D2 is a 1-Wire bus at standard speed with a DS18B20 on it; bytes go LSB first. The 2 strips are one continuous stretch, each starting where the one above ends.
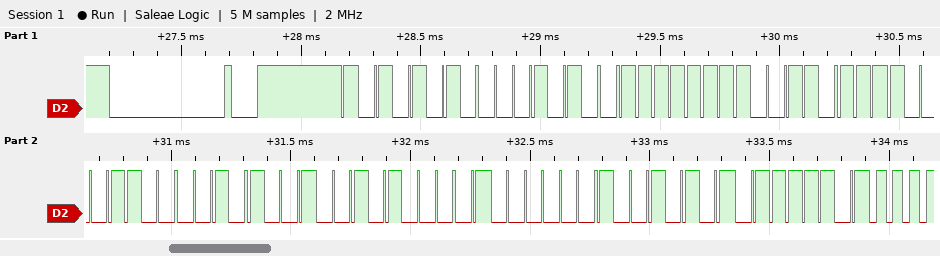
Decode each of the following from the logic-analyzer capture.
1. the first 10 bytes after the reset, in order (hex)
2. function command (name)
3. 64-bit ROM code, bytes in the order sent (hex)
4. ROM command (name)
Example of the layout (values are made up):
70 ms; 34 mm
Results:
55 28 FF EC 31 94 14 02 A9 BE; Read Scratchpad; 28 FF EC 31 94 14 02 A9; Match ROM
